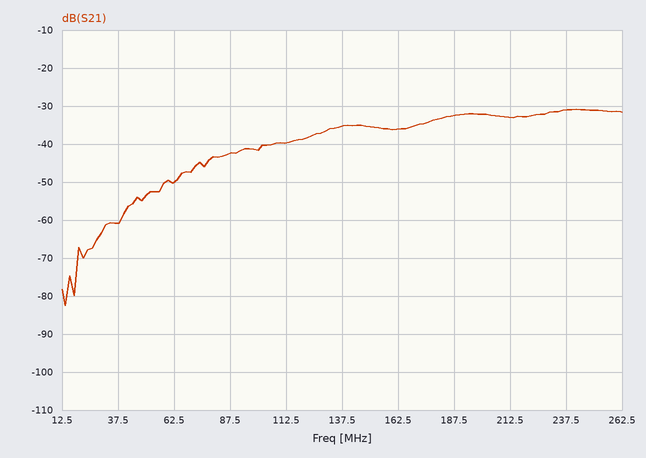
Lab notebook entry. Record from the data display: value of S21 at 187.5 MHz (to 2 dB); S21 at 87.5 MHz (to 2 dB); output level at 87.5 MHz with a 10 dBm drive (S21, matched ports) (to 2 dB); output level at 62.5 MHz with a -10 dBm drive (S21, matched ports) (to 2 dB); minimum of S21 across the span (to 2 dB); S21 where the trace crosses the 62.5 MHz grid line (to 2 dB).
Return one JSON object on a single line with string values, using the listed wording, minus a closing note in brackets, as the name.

{"value of S21 at 187.5 MHz": "-32 dB", "S21 at 87.5 MHz": "-42 dB", "output level at 87.5 MHz with a 10 dBm drive (S21, matched ports)": "-32 dBm", "output level at 62.5 MHz with a -10 dBm drive (S21, matched ports)": "-60 dBm", "minimum of S21 across the span": "-82 dB", "S21 where the trace crosses the 62.5 MHz grid line": "-50 dB"}
